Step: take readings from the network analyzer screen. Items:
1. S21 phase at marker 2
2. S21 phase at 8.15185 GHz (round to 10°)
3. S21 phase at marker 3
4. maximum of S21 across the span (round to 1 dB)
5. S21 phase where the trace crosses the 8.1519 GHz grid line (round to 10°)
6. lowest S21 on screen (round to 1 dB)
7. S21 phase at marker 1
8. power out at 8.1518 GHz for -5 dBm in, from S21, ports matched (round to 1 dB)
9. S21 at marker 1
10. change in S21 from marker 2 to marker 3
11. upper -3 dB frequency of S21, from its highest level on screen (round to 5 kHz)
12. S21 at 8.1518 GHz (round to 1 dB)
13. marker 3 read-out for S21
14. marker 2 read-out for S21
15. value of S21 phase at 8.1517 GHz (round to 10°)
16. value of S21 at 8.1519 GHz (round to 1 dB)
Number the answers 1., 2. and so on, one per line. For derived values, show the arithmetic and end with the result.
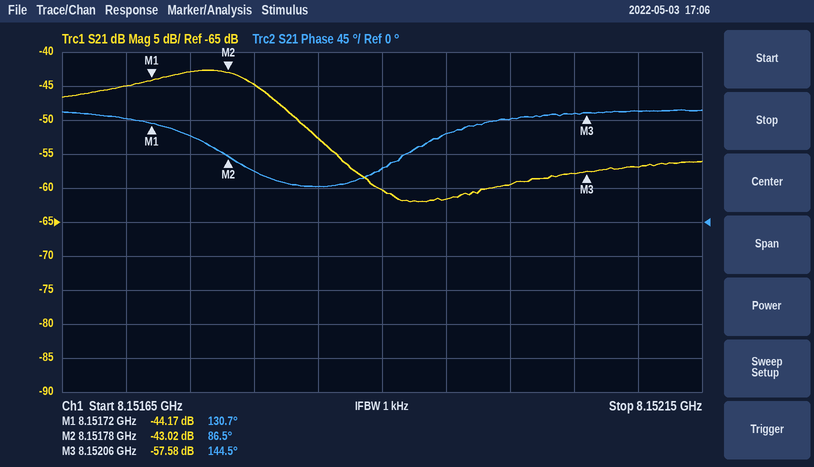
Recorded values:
1. 86.5°
2. 50°
3. 144.5°
4. -43 dB
5. 70°
6. -62 dB
7. 130.7°
8. -5 dBm + (-45 dB) = -50 dBm
9. -44.17 dB
10. -57.58 − (-43.02) = -14.56 dB
11. 8.151805 GHz
12. -45 dB
13. -57.58 dB
14. -43.02 dB
15. 140°
16. -60 dB
